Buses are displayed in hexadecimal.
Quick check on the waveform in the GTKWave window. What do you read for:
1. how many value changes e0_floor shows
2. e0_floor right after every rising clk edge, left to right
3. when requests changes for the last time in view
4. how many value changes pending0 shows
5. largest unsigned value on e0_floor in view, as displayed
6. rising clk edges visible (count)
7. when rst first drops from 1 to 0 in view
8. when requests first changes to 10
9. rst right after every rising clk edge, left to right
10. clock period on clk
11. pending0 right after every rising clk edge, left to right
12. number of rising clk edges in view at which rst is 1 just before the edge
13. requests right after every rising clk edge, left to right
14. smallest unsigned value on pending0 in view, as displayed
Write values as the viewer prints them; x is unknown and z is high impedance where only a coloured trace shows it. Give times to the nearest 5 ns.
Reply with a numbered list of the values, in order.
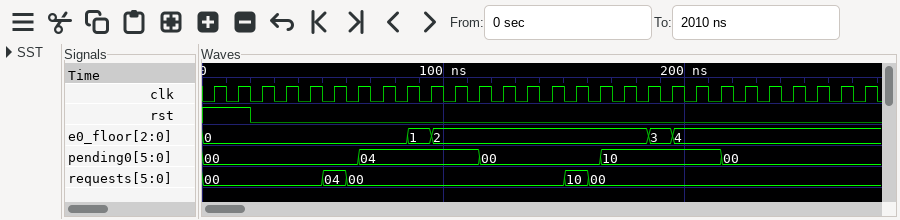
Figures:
1. 4
2. 0, 0, 0, 0, 0, 0, 0, 0, 1, 2, 2, 2, 2, 2, 2, 2, 2, 2, 3, 4, 4, 4, 4, 4, 4, 4, 4, 4
3. 160 ns
4. 4
5. 4
6. 28
7. 20 ns
8. 150 ns
9. 1 1 0 0 0 0 0 0 0 0 0 0 0 0 0 0 0 0 0 0 0 0 0 0 0 0 0 0
10. 10 ns
11. 00, 00, 00, 00, 00, 00, 04, 04, 04, 04, 04, 00, 00, 00, 00, 00, 10, 10, 10, 10, 10, 00, 00, 00, 00, 00, 00, 00
12. 2
13. 00, 00, 00, 00, 00, 04, 00, 00, 00, 00, 00, 00, 00, 00, 00, 10, 00, 00, 00, 00, 00, 00, 00, 00, 00, 00, 00, 00
14. 00
